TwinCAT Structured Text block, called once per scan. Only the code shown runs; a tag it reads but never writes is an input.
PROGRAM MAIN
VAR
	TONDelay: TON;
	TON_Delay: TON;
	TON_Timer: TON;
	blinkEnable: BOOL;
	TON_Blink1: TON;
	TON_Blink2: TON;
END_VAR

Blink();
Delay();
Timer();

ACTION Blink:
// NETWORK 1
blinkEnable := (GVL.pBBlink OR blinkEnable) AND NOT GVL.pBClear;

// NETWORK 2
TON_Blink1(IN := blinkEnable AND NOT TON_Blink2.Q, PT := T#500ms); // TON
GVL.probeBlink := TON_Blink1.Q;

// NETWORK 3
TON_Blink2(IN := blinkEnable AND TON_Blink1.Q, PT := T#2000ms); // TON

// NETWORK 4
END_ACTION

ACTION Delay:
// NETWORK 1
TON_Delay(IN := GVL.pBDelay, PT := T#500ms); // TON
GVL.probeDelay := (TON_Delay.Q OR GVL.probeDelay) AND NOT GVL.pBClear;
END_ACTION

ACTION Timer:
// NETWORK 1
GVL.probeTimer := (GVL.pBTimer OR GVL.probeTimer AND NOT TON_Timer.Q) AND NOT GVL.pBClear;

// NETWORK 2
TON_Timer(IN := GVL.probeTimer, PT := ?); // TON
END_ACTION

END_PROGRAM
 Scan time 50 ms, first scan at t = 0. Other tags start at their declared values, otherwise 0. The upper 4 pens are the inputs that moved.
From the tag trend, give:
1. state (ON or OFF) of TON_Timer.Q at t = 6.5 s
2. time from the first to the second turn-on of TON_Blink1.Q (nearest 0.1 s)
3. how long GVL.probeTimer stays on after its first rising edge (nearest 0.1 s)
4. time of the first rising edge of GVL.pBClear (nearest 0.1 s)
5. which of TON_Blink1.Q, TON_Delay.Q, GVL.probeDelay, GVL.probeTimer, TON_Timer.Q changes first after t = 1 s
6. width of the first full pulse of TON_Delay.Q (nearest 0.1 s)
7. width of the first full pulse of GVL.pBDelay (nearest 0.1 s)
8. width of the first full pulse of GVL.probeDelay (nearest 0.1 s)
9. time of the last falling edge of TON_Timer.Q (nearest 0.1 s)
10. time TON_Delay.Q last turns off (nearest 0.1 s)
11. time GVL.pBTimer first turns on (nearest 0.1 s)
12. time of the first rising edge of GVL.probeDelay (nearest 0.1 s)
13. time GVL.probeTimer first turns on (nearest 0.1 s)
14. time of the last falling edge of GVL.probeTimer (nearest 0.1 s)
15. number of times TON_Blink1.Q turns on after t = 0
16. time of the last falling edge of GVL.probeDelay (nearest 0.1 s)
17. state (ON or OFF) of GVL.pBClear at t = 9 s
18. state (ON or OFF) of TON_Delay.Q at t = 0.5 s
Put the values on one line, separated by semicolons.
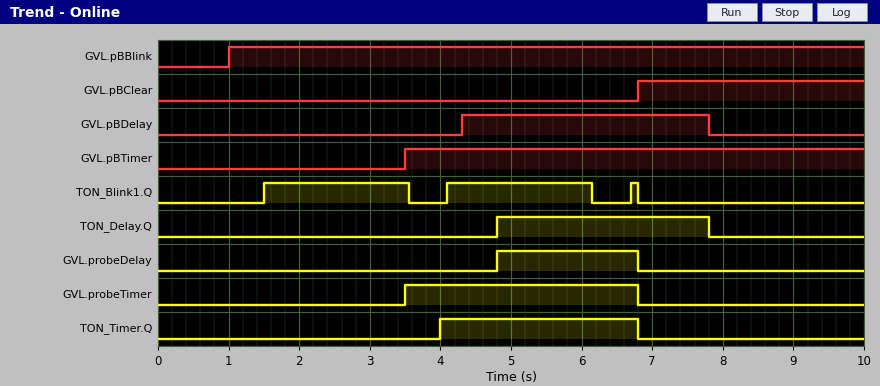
ON; 2.6 s; 3.3 s; 6.8 s; TON_Blink1.Q; 3.0 s; 3.5 s; 2.0 s; 6.8 s; 7.8 s; 3.5 s; 4.8 s; 3.5 s; 6.8 s; 3; 6.8 s; ON; OFF
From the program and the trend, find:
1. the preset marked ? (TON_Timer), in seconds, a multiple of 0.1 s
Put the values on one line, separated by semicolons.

0.5 s
